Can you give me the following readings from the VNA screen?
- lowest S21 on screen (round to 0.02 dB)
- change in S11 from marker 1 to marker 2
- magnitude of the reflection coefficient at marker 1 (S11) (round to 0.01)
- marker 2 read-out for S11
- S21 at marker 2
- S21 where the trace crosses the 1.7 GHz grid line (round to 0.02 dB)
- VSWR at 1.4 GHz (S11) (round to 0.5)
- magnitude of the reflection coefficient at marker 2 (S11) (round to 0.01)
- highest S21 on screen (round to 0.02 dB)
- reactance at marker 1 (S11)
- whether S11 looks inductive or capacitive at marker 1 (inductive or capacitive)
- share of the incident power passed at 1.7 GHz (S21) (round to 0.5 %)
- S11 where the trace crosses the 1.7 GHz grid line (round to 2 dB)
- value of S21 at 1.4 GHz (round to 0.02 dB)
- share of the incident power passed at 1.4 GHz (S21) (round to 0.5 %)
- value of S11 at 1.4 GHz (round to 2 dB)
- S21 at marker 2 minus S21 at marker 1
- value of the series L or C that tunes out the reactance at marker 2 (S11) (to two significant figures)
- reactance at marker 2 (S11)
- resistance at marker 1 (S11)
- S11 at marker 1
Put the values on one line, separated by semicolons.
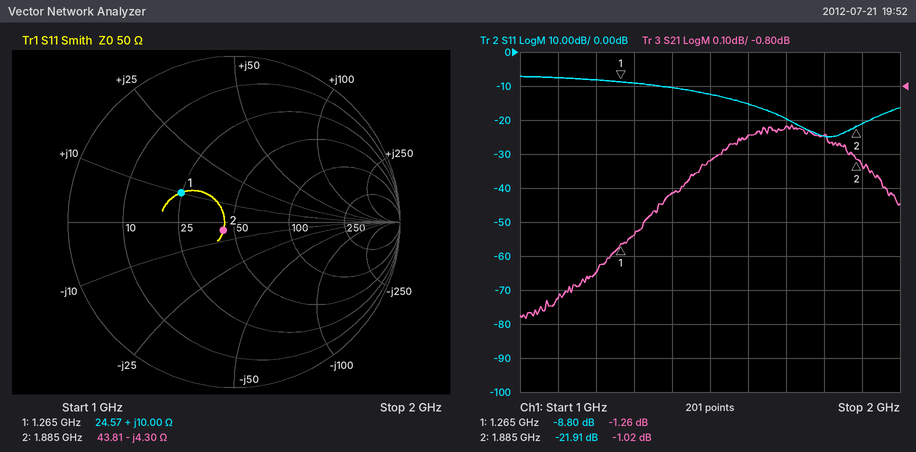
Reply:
-1.48 dB; -13.11 dB; 0.36; -21.91 dB; -1.02 dB; -0.92 dB; 2.0; 0.08; -0.92 dB; +10.00 Ω; inductive; 81.0 %; -20 dB; -1.12 dB; 77.5 %; -10 dB; 0.24 dB; 360 pH; -4.30 Ω; 24.57 Ω; -8.80 dB
